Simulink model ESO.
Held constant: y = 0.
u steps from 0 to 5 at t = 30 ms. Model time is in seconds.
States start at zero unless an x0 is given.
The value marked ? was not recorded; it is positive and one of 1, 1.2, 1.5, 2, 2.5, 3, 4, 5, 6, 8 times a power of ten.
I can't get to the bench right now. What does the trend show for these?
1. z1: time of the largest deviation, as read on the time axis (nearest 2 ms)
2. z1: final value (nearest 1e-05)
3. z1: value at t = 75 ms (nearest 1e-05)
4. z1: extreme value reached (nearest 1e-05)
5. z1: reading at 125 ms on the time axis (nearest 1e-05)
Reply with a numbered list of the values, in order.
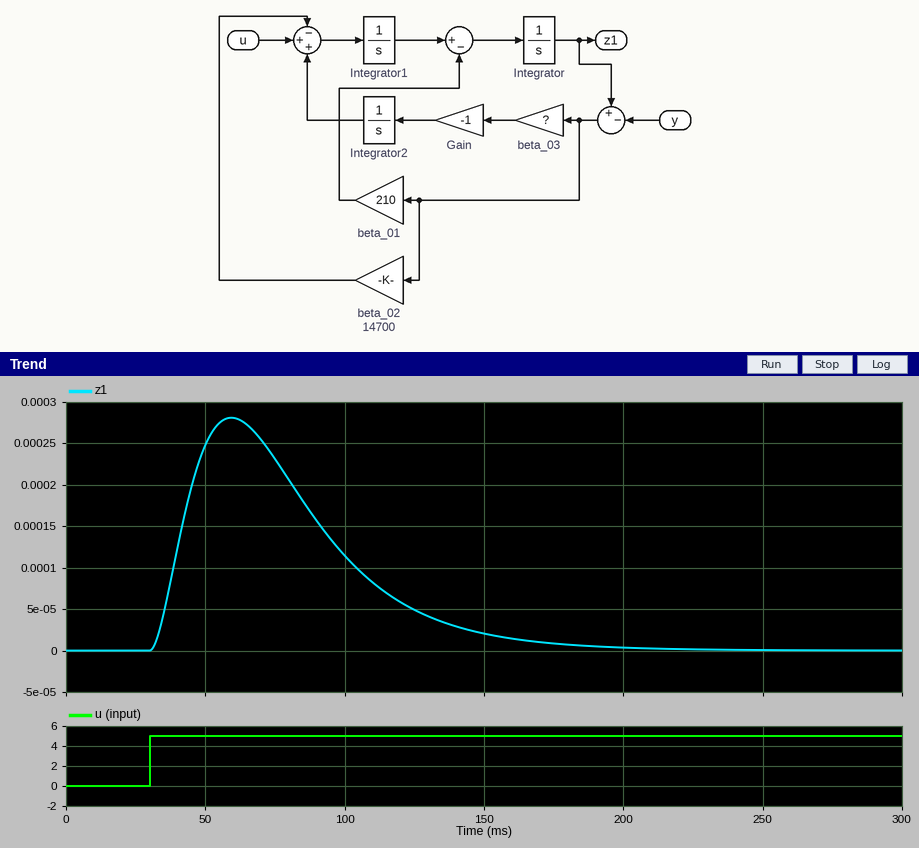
1. 60 ms
2. 0.00000
3. 0.00023
4. 0.00028
5. 0.00005
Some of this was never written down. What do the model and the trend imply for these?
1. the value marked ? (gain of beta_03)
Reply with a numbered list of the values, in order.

1. 300000
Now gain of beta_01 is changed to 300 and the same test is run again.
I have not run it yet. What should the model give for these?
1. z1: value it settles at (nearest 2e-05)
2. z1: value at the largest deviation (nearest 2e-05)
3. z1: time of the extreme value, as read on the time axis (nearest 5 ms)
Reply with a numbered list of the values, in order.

1. 0.00000
2. 0.00024
3. 65 ms
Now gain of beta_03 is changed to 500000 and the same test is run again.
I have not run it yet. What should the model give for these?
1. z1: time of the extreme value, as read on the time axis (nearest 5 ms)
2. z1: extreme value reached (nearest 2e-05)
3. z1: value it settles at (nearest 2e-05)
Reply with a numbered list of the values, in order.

1. 55 ms
2. 0.00026
3. 0.00000
